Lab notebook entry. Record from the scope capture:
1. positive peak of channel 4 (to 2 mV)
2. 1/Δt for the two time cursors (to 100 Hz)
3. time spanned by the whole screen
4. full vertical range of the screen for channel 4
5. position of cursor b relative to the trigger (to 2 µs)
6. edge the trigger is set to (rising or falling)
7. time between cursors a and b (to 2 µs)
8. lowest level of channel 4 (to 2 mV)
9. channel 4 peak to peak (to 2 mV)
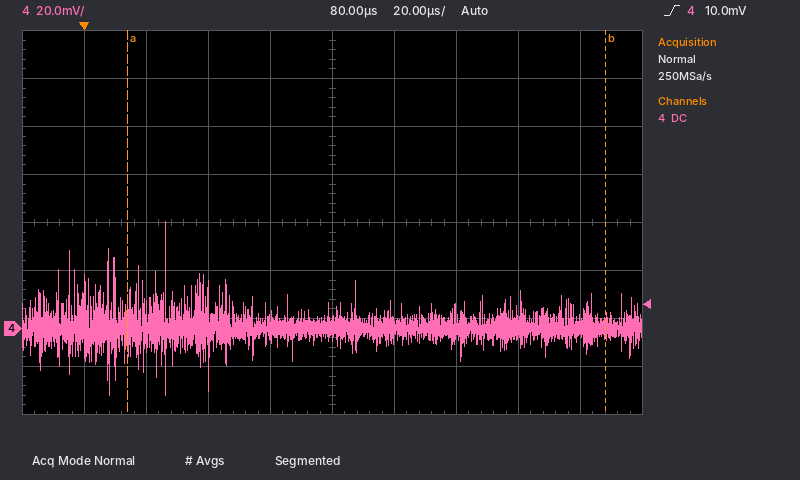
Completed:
44 mV
6.5 kHz
200 µs
160 mV
+168 µs
rising
154 µs
-28 mV
72 mV
